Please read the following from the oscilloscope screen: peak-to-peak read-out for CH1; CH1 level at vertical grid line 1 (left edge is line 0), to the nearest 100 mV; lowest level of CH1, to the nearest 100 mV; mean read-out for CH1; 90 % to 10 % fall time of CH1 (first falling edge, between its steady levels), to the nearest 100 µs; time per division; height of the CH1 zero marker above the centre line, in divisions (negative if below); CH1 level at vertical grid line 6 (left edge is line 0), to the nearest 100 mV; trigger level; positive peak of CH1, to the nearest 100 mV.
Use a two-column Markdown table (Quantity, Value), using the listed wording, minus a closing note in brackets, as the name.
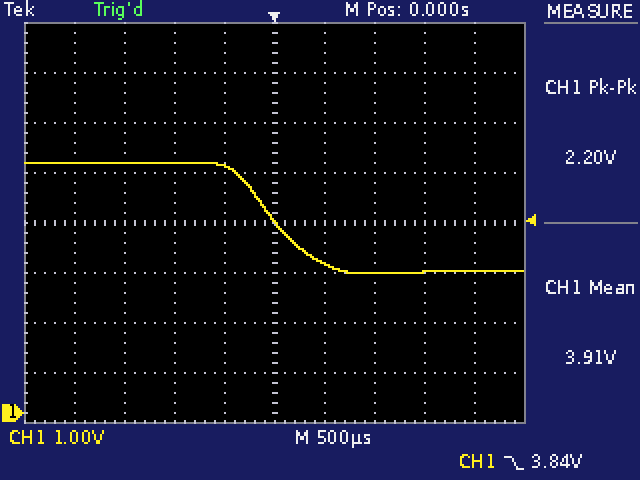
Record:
| Quantity | Value |
|---|---|
| peak-to-peak read-out for CH1 | 2.20 V |
| CH1 level at vertical grid line 1 (left edge is line 0), to the nearest 100 mV | 5.0 V |
| lowest level of CH1, to the nearest 100 mV | 2.8 V |
| mean read-out for CH1 | 3.91 V |
| 90 % to 10 % fall time of CH1 (first falling edge, between its steady levels), to the nearest 100 µs | 800 µs |
| time per division | 500 µs |
| height of the CH1 zero marker above the centre line, in divisions | -3.8 div |
| CH1 level at vertical grid line 6 (left edge is line 0), to the nearest 100 mV | 3.0 V |
| trigger level | 3.84 V |
| positive peak of CH1, to the nearest 100 mV | 5.0 V |
